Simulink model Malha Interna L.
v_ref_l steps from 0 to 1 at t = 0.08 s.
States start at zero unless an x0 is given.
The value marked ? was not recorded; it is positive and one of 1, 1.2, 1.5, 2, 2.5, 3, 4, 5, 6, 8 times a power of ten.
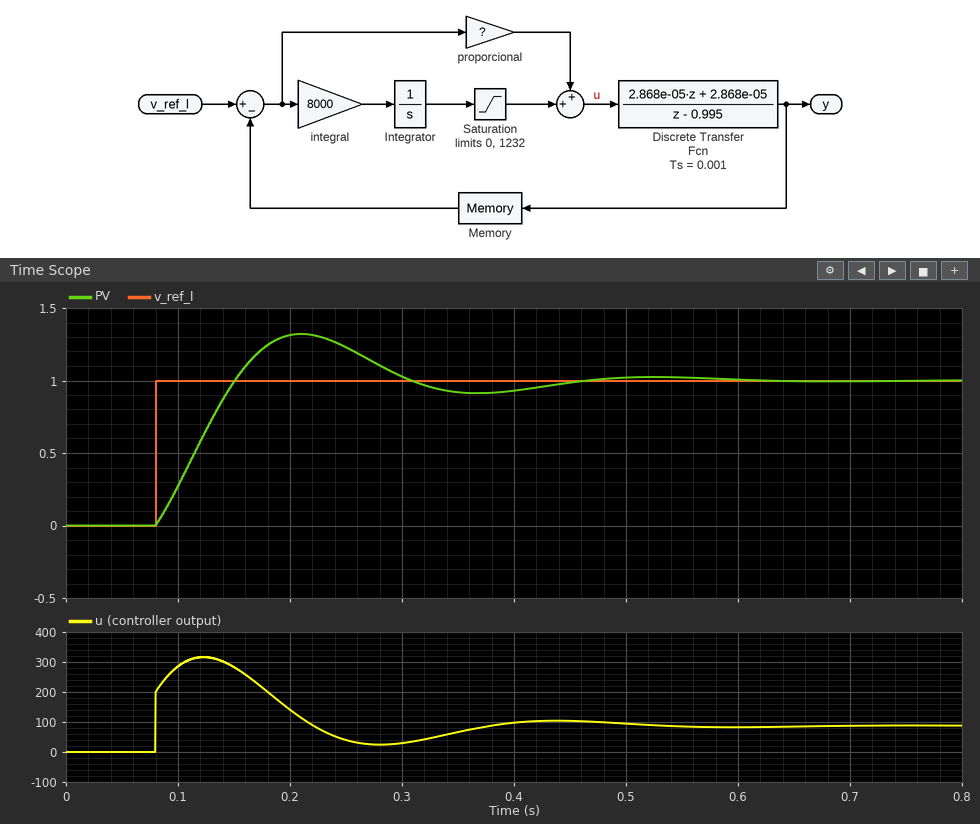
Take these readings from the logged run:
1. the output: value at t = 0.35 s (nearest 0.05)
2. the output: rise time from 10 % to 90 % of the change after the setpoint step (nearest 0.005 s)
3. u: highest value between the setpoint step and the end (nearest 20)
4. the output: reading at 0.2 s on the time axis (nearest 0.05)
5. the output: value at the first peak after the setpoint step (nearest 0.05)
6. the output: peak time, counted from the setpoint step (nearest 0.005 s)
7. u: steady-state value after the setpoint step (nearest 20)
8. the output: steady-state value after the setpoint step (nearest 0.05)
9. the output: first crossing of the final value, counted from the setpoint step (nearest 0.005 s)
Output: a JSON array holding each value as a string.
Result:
["0.90", "0.055 s", "320", "1.30", "1.30", "0.130 s", "80", "1.00", "0.070 s"]
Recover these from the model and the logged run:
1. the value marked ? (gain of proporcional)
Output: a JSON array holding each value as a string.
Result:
["200"]
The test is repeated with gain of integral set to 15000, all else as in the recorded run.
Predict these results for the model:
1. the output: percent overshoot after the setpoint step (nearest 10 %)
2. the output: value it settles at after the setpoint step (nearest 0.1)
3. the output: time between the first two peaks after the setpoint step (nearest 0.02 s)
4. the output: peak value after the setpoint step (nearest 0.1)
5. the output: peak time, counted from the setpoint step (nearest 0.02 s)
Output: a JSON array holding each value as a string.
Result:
["40 %", "1.0", "0.24 s", "1.4", "0.10 s"]
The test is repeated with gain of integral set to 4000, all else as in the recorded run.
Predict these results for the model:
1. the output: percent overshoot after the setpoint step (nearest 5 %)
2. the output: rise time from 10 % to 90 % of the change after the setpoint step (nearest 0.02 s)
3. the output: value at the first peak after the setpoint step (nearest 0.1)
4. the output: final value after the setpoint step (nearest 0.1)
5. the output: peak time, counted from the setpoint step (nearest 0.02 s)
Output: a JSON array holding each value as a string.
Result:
["20 %", "0.08 s", "1.2", "1.0", "0.18 s"]
